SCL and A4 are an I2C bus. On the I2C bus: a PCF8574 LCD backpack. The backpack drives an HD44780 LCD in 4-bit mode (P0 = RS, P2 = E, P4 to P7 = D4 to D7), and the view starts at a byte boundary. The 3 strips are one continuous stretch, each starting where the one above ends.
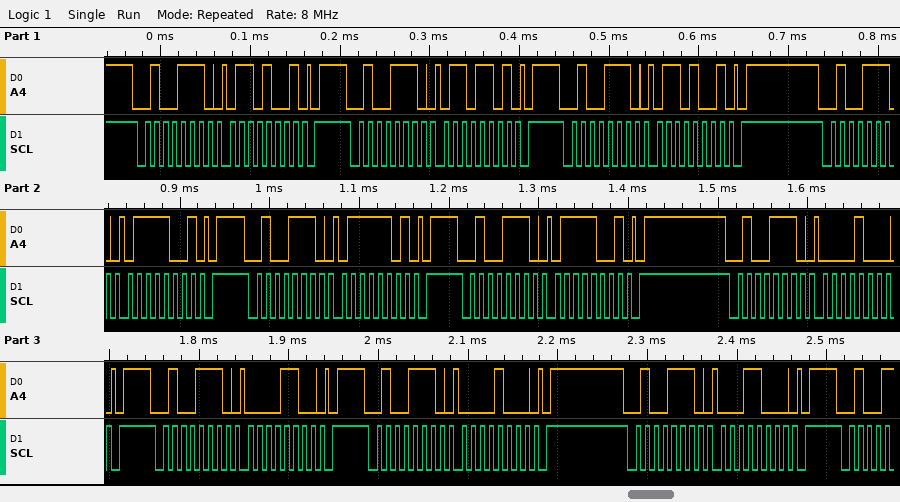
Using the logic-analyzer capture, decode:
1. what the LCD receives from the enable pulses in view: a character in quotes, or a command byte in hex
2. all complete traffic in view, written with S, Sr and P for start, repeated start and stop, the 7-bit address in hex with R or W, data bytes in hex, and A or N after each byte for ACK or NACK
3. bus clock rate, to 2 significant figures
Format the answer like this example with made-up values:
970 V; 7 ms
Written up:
'g'; S 27W A 69 A P S 27W A 6D A P S 27W A 69 A P S 27W A 79 A P S 27W A 7D A P S 27W A 79 A P S 27W A 08 A P S 27W A 0C A P S 27W A 08 A P S 27W A 18 A P; 100 kHz
